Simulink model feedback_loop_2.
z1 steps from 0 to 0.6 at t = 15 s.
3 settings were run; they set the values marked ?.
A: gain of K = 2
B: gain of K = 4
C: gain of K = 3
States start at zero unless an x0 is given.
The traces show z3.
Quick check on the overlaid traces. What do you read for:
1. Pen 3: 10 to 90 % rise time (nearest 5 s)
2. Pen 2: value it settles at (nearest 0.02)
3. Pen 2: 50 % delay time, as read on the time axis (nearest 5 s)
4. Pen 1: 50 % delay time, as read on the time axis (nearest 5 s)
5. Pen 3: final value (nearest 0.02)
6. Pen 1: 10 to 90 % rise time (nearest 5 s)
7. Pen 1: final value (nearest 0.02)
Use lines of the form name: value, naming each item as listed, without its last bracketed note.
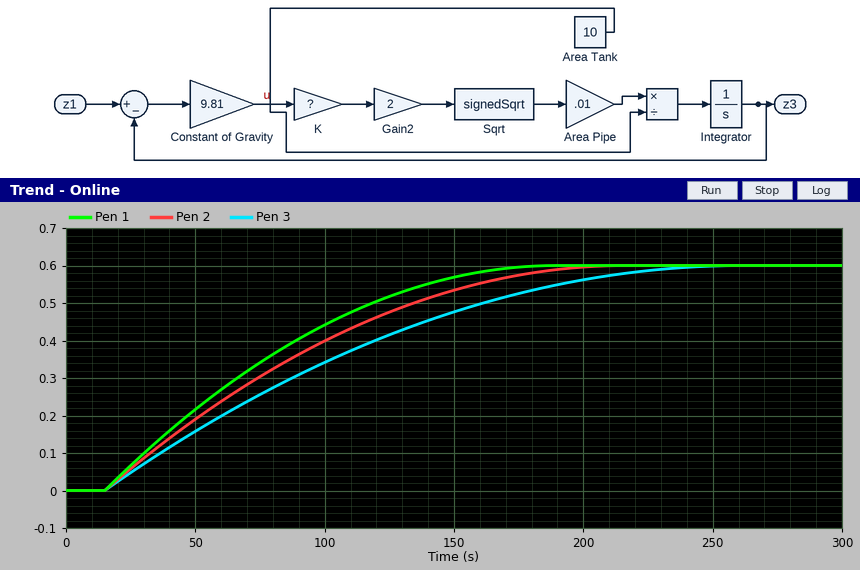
Pen 3: 10 to 90 % rise time: 155 s
Pen 2: value it settles at: 0.60
Pen 2: 50 % delay time, as read on the time axis: 75 s
Pen 1: 50 % delay time, as read on the time axis: 65 s
Pen 3: final value: 0.60
Pen 1: 10 to 90 % rise time: 110 s
Pen 1: final value: 0.60
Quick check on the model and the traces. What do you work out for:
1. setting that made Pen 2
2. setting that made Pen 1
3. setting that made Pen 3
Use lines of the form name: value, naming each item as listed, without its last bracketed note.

setting that made Pen 2: C
setting that made Pen 1: B
setting that made Pen 3: A
